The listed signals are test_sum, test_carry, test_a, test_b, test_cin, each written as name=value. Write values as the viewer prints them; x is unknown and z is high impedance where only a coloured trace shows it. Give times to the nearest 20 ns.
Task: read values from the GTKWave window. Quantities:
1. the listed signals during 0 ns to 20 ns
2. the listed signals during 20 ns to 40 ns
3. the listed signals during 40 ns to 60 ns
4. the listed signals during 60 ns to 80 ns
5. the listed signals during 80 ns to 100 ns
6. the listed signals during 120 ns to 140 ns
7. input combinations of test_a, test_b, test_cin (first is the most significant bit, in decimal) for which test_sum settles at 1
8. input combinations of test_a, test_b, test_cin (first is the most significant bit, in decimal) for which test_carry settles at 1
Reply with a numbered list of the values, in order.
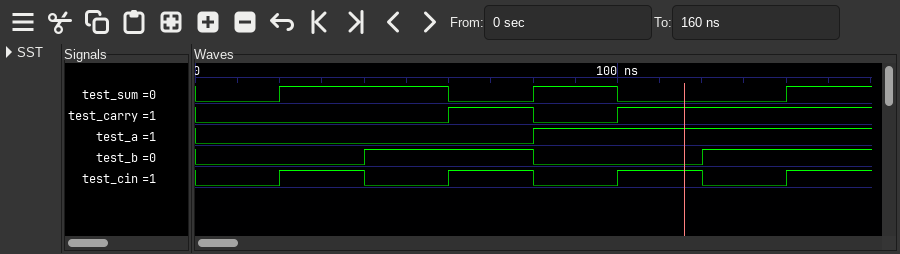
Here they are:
1. test_sum=0, test_carry=0, test_a=0, test_b=0, test_cin=0
2. test_sum=1, test_carry=0, test_a=0, test_b=0, test_cin=1
3. test_sum=1, test_carry=0, test_a=0, test_b=1, test_cin=0
4. test_sum=0, test_carry=1, test_a=0, test_b=1, test_cin=1
5. test_sum=1, test_carry=0, test_a=1, test_b=0, test_cin=0
6. test_sum=0, test_carry=1, test_a=1, test_b=1, test_cin=0
7. 1, 2, 4, 7
8. 3, 5, 6, 7
